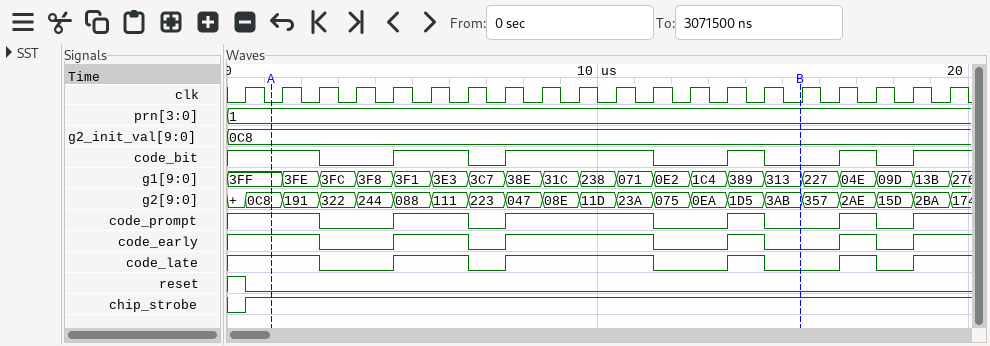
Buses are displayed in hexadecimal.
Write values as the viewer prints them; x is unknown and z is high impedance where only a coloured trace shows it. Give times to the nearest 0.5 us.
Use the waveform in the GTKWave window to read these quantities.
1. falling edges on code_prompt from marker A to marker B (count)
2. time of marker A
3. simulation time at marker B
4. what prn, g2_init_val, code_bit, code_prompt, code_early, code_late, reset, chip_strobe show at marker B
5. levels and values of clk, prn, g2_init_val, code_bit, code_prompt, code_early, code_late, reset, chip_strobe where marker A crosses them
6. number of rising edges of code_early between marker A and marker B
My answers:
4
1 us
15.5 us
prn=1, g2_init_val=0C8, code_bit=0, code_prompt=0, code_early=0, code_late=0, reset=0, chip_strobe=1
clk=0, prn=1, g2_init_val=0C8, code_bit=1, code_prompt=1, code_early=1, code_late=1, reset=0, chip_strobe=1
3
